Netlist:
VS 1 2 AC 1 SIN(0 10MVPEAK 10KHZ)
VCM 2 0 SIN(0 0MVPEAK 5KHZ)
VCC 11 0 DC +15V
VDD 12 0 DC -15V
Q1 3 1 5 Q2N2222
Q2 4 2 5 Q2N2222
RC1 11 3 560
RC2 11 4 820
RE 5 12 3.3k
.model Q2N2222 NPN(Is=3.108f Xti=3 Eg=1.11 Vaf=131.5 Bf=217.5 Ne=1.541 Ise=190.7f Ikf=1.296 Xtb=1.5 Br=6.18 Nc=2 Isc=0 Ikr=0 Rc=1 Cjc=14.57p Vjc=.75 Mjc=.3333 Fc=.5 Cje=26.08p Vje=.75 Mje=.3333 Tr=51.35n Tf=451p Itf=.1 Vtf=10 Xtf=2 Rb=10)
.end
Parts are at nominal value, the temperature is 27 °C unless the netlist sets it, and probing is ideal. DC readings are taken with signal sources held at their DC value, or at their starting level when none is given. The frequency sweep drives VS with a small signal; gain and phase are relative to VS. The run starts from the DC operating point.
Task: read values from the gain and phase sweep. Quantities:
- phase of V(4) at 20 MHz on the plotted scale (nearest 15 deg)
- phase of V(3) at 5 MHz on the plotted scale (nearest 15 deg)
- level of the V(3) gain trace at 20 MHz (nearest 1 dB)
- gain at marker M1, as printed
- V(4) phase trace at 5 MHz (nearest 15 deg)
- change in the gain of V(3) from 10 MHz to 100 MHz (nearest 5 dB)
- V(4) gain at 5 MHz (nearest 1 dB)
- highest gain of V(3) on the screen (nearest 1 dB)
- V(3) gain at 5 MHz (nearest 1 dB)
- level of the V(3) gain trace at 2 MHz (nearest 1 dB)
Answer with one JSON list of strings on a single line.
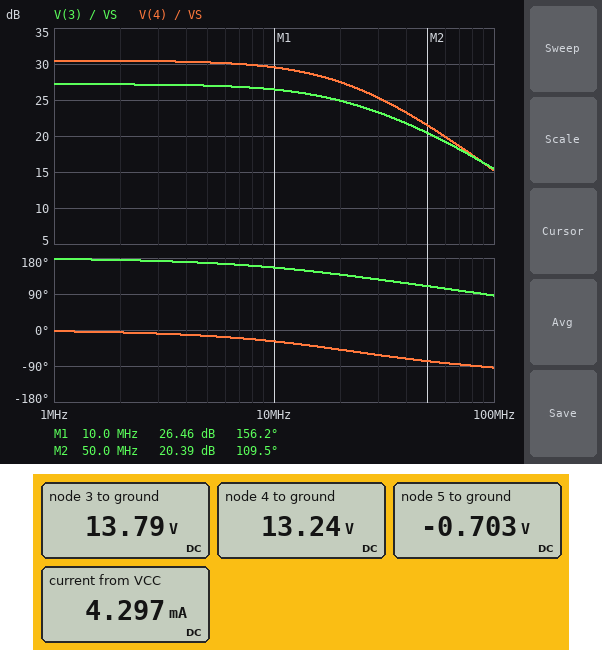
["-45 deg", "165 deg", "25 dB", "26.46 dB", "-15 deg", "-10 dB", "30 dB", "27 dB", "27 dB", "27 dB"]
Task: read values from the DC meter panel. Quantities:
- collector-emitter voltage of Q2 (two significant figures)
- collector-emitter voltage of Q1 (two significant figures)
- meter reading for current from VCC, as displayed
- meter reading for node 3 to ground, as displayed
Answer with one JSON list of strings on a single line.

["14 V", "14 V", "4.297 mA", "13.79 V"]
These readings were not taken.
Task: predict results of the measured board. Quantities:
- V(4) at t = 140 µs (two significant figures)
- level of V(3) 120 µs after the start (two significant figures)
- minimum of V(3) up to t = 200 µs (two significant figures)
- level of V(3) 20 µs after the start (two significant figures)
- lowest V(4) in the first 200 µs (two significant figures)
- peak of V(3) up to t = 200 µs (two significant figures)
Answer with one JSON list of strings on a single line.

["13 V", "14 V", "14 V", "14 V", "13 V", "14 V"]
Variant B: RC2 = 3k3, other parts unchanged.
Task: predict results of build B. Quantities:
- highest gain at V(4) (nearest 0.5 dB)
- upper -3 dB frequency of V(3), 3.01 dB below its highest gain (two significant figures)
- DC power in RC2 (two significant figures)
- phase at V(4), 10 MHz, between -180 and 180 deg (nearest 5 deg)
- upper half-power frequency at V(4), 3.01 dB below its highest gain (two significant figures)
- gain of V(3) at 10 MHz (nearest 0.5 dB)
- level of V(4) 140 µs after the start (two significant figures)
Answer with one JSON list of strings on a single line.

["42.5 dB", "15 MHz", "15 mW", "-65 deg", "5.3 MHz", "24.5 dB", "8.8 V"]
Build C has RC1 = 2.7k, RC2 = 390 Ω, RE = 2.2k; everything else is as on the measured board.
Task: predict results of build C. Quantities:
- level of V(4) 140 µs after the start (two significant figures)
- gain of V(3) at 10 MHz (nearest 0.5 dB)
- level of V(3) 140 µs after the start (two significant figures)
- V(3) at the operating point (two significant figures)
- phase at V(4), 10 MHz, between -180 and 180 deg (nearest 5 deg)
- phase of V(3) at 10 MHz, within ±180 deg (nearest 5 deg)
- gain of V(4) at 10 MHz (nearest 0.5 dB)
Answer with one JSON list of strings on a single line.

["14 V", "37.5 dB", "5.6 V", "6.5 V", "-25 deg", "115 deg", "24.5 dB"]
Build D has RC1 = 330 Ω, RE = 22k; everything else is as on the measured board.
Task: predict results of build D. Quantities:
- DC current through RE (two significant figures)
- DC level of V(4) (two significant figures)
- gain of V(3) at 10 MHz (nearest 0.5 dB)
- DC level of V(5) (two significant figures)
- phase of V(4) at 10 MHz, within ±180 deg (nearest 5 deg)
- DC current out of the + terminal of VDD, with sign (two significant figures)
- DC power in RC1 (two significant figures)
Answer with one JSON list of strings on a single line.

["650 µA", "15 V", "6.0 dB", "-650 mV", "-20 deg", "-650 µA", "34 µW"]
